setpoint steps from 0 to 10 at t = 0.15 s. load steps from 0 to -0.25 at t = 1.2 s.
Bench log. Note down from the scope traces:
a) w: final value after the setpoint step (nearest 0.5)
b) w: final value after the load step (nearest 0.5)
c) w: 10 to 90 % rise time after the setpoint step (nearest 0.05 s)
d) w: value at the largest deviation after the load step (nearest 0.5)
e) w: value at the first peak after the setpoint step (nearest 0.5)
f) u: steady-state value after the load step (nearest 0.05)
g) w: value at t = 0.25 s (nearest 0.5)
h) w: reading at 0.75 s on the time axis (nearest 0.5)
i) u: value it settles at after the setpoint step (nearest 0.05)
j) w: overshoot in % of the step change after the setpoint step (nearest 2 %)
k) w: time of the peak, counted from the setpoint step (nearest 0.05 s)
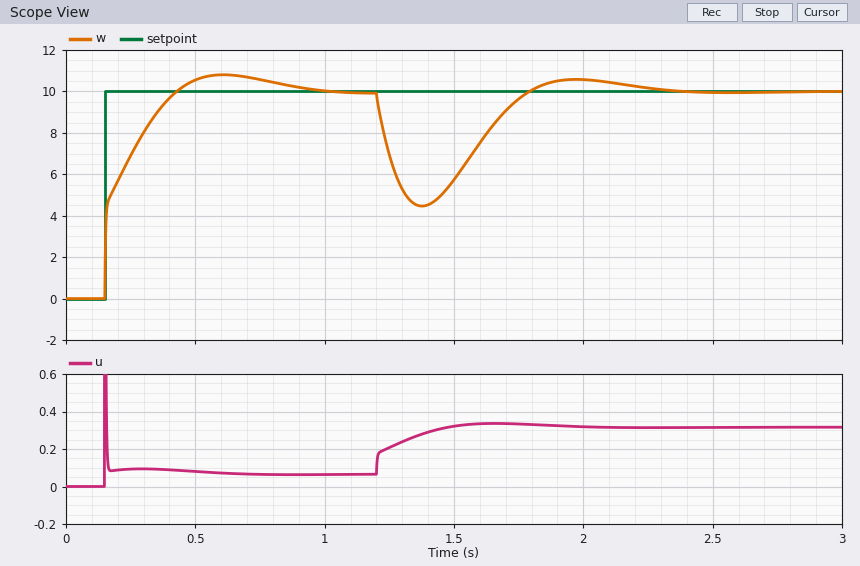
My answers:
10.0
10.0
0.20 s
4.5
11.0
0.30
7.0
10.5
0.05
8 %
0.45 s
